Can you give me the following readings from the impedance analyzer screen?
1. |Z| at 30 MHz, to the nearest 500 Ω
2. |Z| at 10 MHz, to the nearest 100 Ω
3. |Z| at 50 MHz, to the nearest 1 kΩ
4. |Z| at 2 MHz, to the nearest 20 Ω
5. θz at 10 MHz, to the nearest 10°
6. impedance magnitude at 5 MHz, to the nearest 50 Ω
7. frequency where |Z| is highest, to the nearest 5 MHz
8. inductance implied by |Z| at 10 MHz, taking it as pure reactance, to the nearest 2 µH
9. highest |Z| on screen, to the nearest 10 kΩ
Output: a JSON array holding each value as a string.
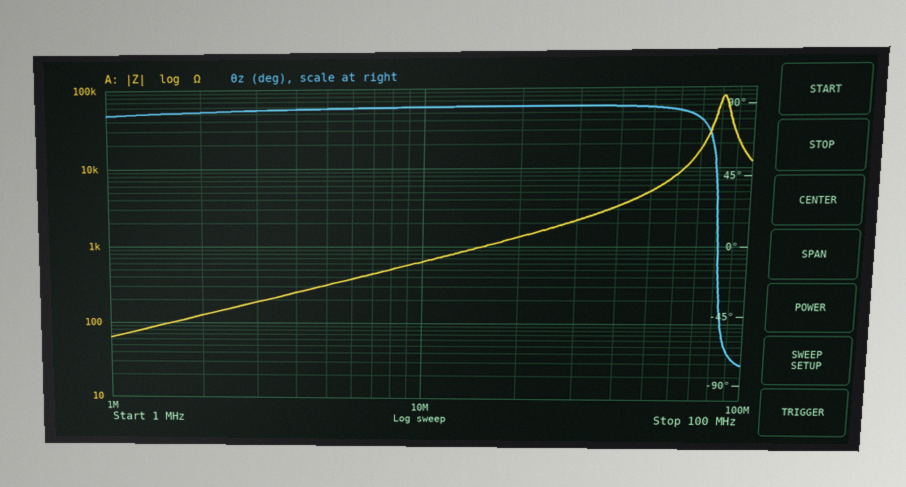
["2.0 kΩ", "600 Ω", "5 kΩ", "120 Ω", "90°", "300 Ω", "80 MHz", "10 µH", "80 kΩ"]
